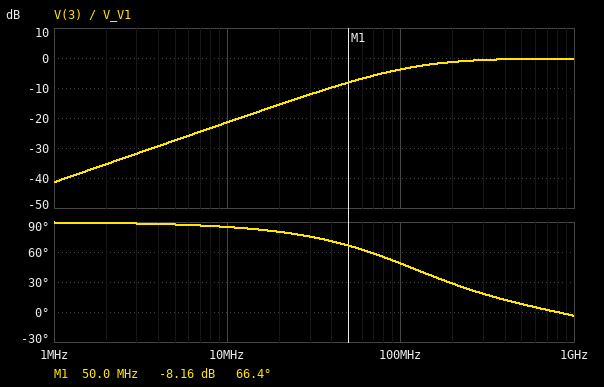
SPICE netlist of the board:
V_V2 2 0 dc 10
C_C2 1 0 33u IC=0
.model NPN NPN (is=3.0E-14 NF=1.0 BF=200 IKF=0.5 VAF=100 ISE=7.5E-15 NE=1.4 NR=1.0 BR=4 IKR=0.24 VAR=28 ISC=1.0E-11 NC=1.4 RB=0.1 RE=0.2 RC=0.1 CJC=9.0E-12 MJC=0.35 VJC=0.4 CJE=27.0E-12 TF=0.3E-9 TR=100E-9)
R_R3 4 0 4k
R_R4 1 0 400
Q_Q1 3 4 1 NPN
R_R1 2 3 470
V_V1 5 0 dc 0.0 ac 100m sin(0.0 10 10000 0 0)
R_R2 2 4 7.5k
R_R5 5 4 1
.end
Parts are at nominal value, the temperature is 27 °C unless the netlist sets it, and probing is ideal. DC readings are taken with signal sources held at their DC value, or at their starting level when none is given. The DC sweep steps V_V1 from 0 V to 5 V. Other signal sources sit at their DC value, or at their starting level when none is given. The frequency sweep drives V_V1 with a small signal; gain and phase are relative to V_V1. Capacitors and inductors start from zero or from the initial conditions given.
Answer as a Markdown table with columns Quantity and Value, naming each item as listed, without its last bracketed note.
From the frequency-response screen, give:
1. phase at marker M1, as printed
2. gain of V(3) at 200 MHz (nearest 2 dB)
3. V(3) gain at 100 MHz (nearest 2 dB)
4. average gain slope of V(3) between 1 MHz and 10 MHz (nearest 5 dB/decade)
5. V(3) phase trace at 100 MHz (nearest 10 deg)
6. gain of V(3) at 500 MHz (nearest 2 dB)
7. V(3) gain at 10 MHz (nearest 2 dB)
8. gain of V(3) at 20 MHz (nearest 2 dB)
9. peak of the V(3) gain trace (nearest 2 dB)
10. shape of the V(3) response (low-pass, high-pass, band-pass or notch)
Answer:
| Quantity | Value |
|---|---|
| phase at marker M1, as printed | 66.4 deg |
| gain of V(3) at 200 MHz | -2 dB |
| V(3) gain at 100 MHz | -4 dB |
| average gain slope of V(3) between 1 MHz and 10 MHz | 20 dB/decade |
| V(3) phase trace at 100 MHz | 50 deg |
| gain of V(3) at 500 MHz | 0 dB |
| V(3) gain at 10 MHz | -22 dB |
| gain of V(3) at 20 MHz | -16 dB |
| peak of the V(3) gain trace | 0 dB |
| shape of the V(3) response | high-pass |
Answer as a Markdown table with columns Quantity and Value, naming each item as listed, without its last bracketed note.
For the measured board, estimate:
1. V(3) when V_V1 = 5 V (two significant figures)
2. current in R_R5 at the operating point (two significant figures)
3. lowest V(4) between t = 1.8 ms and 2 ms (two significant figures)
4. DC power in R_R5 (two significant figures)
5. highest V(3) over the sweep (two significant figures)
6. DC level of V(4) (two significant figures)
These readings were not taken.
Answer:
| Quantity | Value |
|---|---|
| V(3) when V_V1 = 5 V | 5.0 V |
| current in R_R5 at the operating point | 1.3 mA |
| lowest V(4) between t = 1.8 ms and 2 ms | -10 V |
| DC power in R_R5 | 1.8 µW |
| highest V(3) over the sweep | 10 V |
| DC level of V(4) | 1.3 mV |
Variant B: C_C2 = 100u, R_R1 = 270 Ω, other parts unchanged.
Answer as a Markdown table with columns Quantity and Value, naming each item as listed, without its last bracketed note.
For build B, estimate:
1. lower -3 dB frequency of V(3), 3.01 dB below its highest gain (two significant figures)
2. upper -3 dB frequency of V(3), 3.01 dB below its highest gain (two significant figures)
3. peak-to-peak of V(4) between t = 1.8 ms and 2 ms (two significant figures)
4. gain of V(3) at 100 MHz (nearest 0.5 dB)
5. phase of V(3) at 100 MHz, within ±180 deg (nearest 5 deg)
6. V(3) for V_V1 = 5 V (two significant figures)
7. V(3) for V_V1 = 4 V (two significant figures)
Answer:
| Quantity | Value |
|---|---|
| lower -3 dB frequency of V(3), 3.01 dB below its highest gain | 190 MHz |
| upper -3 dB frequency of V(3), 3.01 dB below its highest gain | 5.1 GHz |
| peak-to-peak of V(4) between t = 1.8 ms and 2 ms | 19 V |
| gain of V(3) at 100 MHz | -7.0 dB |
| phase of V(3) at 100 MHz, within ±180 deg | 65 deg |
| V(3) for V_V1 = 5 V | 7.1 V |
| V(3) for V_V1 = 4 V | 7.8 V |
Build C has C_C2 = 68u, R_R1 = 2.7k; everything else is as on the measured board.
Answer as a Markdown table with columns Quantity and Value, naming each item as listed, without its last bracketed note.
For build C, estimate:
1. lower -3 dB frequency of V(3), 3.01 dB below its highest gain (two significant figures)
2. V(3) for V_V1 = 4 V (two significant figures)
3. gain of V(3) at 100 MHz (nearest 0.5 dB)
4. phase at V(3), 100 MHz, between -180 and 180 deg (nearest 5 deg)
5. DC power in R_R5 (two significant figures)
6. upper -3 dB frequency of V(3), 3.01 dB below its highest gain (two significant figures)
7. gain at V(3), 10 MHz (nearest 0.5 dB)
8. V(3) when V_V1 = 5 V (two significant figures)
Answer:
| Quantity | Value |
|---|---|
| lower -3 dB frequency of V(3), 3.01 dB below its highest gain | 20 MHz |
| V(3) for V_V1 = 4 V | 3.3 V |
| gain of V(3) at 100 MHz | 0 dB |
| phase at V(3), 100 MHz, between -180 and 180 deg | 10 deg |
| DC power in R_R5 | 1.8 µW |
| upper -3 dB frequency of V(3), 3.01 dB below its highest gain | 4.7 GHz |
| gain at V(3), 10 MHz | -7.0 dB |
| V(3) when V_V1 = 5 V | 4.3 V |
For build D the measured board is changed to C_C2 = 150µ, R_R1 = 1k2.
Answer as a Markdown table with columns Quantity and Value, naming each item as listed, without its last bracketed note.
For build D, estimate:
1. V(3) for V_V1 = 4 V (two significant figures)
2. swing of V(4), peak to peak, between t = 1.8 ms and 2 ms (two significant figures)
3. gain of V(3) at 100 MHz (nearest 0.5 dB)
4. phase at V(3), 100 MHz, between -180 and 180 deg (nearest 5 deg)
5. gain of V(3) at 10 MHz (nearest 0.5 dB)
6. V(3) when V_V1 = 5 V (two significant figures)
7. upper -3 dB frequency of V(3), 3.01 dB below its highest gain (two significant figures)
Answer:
| Quantity | Value |
|---|---|
| V(3) for V_V1 = 4 V | 3.3 V |
| swing of V(4), peak to peak, between t = 1.8 ms and 2 ms | 19 V |
| gain of V(3) at 100 MHz | -1.0 dB |
| phase at V(3), 100 MHz, between -180 and 180 deg | 25 deg |
| gain of V(3) at 10 MHz | -13.5 dB |
| V(3) when V_V1 = 5 V | 4.3 V |
| upper -3 dB frequency of V(3), 3.01 dB below its highest gain | 4.7 GHz |
